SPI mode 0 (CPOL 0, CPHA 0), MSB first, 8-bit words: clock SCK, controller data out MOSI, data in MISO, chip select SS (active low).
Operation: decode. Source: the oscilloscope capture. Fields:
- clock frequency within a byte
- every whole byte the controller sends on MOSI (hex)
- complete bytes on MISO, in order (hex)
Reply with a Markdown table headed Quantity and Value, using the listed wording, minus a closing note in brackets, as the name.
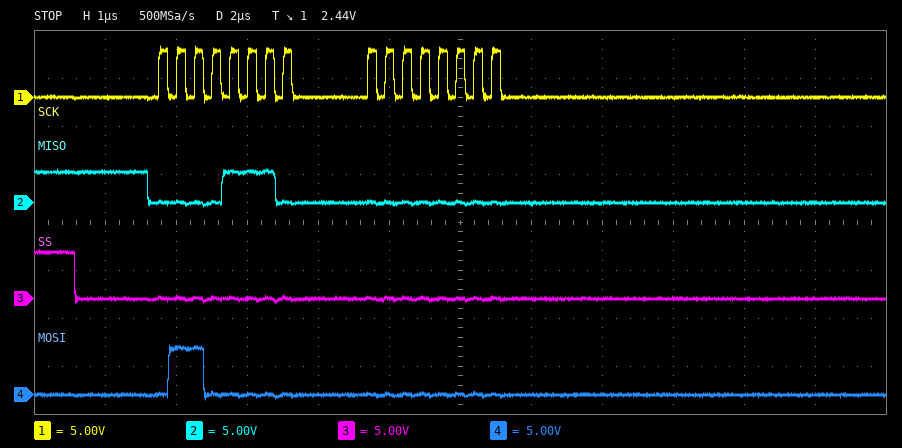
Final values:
| Quantity | Value |
|---|---|
| clock frequency within a byte | 4 MHz |
| every whole byte the controller sends on MOSI | 0x60 0x00 |
| complete bytes on MISO, in order | 0x0E 0x00 |
